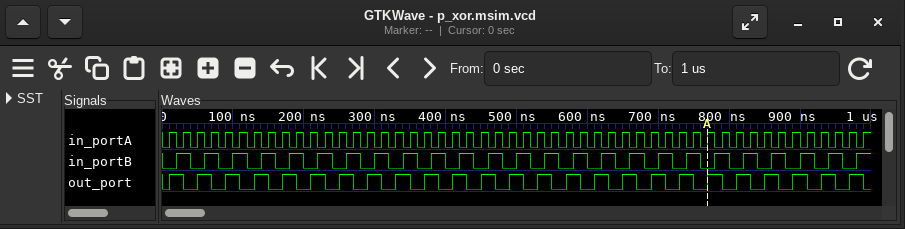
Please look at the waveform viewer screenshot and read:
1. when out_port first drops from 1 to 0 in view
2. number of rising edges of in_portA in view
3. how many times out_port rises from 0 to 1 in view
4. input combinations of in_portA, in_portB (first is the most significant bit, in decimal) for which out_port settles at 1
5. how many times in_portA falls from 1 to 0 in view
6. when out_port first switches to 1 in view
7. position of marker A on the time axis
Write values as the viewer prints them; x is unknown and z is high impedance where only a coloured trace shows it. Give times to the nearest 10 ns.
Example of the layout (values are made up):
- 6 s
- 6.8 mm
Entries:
- 30 ns
- 50
- 25
- 1, 2
- 49
- 10 ns
- 770 ns
